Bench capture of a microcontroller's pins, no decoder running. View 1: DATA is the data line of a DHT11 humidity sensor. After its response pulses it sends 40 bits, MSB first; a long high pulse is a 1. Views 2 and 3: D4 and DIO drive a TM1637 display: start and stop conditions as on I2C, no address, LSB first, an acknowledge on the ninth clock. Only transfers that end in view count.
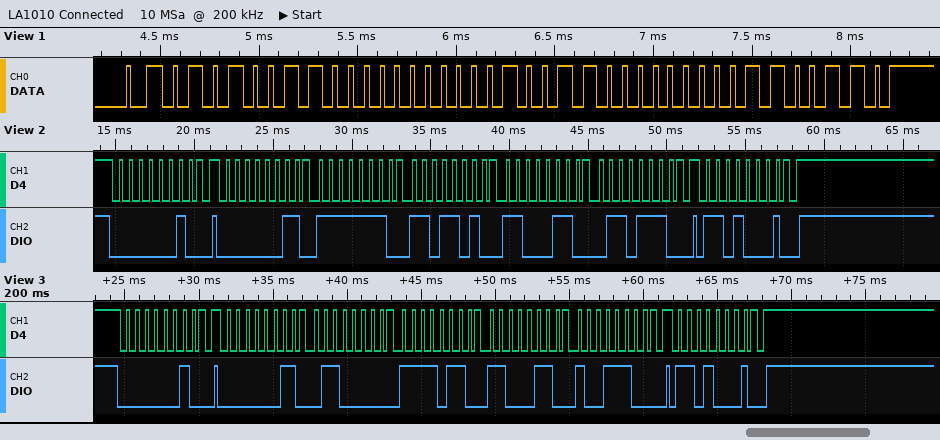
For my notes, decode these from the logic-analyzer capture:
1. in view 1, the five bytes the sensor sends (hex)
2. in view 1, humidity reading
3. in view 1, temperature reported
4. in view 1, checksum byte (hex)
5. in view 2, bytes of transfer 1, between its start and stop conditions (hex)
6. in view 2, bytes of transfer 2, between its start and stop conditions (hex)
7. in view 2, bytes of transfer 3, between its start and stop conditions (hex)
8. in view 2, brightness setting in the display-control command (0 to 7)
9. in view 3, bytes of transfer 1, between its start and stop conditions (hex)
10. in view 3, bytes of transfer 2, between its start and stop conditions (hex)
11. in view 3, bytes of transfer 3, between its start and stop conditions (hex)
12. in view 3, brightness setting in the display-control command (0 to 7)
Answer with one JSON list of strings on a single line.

["53 00 13 00 66", "83 %", "19.0 °C", "0x66", "40", "C0 7F 5B 63 76", "8B", "3", "40", "C0 06 6F 63 39", "8B", "3"]
